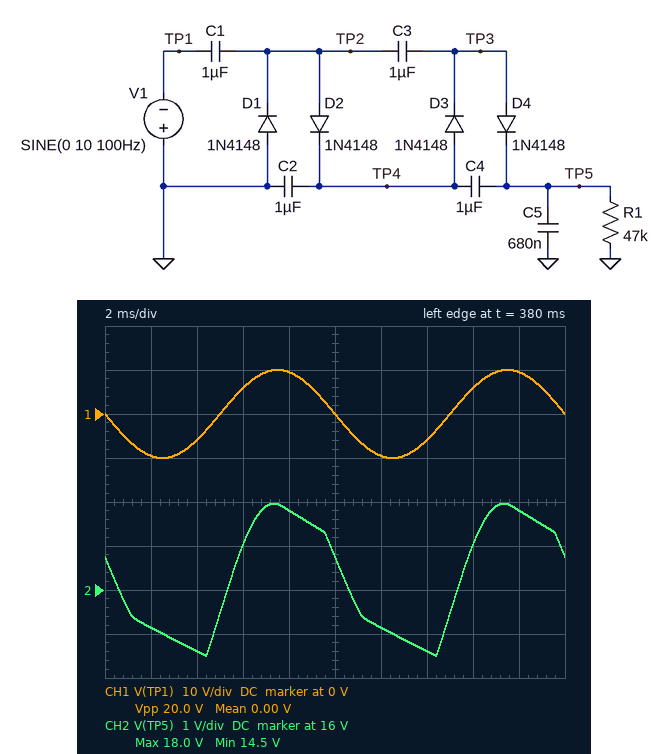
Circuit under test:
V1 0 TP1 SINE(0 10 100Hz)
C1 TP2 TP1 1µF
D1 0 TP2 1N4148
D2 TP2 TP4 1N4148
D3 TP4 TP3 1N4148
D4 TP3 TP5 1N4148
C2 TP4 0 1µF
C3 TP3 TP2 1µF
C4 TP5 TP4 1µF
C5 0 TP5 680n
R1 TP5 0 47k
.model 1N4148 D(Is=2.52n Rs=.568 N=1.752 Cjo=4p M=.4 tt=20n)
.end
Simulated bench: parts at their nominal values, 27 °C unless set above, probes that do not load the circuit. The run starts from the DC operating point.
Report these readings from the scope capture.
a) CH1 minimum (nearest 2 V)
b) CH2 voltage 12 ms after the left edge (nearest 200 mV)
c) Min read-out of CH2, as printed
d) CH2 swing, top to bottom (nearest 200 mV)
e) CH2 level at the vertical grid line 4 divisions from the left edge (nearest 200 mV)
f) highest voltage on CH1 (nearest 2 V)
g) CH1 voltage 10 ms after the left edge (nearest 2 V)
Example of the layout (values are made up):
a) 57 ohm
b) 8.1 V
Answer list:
a) -10 V
b) 15.2 V
c) 14.5 V
d) 3.4 V
e) 17.8 V
f) 10 V
g) 0 V
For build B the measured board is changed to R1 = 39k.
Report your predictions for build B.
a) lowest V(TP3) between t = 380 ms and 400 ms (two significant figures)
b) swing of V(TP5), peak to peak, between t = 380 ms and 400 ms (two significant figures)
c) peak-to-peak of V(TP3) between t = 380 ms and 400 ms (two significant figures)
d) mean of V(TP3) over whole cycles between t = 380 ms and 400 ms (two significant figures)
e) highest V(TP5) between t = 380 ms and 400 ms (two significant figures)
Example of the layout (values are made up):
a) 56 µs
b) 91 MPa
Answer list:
a) 7.8 V
b) 3.7 V
c) 9.1 V
d) 12 V
e) 16 V
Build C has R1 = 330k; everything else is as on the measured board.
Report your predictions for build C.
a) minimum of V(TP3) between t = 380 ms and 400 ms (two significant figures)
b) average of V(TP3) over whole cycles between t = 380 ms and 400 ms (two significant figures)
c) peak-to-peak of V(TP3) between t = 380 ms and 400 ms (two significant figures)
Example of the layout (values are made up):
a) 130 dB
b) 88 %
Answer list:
a) 16 V
b) 24 V
c) 17 V
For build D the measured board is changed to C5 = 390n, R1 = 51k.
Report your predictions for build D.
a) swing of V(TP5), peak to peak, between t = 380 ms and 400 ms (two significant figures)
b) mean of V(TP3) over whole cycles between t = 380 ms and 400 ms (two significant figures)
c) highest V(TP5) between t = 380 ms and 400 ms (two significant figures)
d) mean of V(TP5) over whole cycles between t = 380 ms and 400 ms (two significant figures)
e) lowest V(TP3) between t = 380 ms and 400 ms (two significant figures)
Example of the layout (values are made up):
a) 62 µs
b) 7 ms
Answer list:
a) 4.3 V
b) 14 V
c) 19 V
d) 17 V
e) 8.7 V
